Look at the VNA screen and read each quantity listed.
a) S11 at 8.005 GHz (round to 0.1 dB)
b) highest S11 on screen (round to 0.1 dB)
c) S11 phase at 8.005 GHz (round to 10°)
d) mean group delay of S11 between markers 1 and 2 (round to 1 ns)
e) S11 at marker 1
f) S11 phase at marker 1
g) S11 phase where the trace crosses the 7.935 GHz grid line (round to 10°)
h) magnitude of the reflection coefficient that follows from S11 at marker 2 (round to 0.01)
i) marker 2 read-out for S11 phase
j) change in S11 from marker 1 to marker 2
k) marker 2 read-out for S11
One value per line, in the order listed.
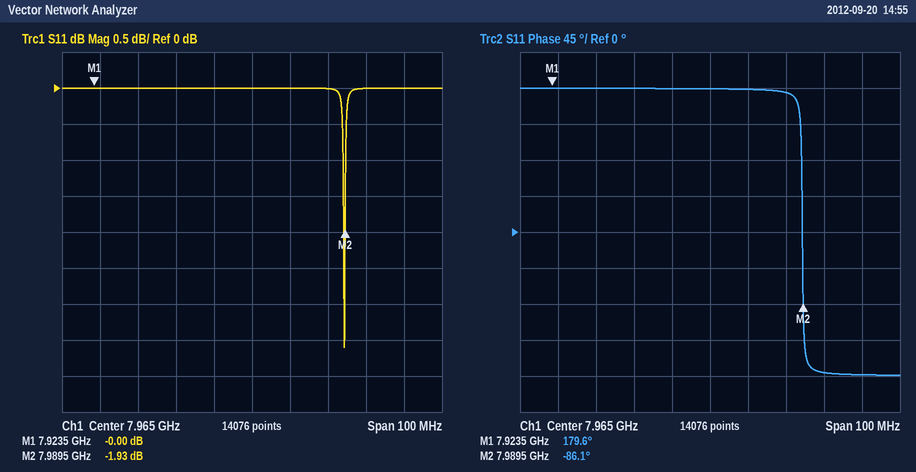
0.0 dB
0.0 dB
-180°
11 ns
-0.00 dB
179.6°
180°
0.80
-86.1°
-1.93 dB
-1.93 dB
